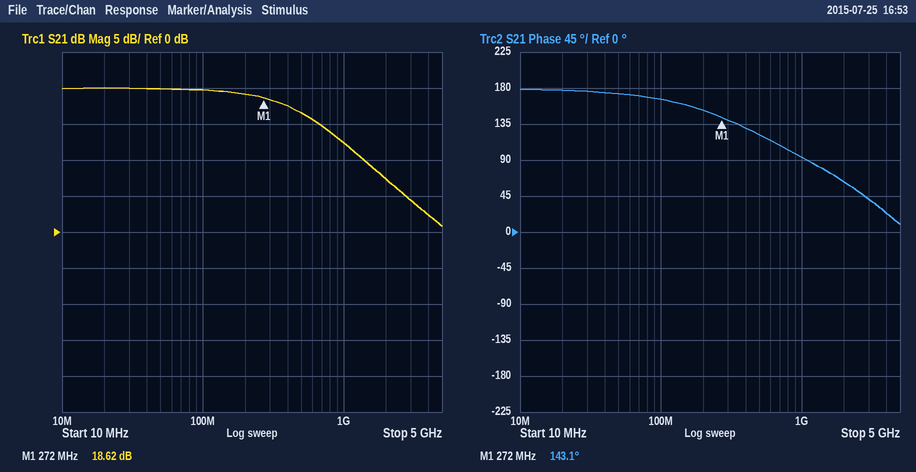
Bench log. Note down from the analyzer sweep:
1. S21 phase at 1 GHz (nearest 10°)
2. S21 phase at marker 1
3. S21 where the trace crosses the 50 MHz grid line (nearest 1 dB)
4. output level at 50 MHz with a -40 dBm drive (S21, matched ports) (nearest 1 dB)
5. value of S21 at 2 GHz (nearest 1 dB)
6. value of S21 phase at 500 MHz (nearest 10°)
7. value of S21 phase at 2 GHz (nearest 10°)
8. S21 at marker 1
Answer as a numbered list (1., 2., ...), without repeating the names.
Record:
1. 90°
2. 143.1°
3. 20 dB
4. -20 dBm
5. 7 dB
6. 120°
7. 60°
8. 18.62 dB
